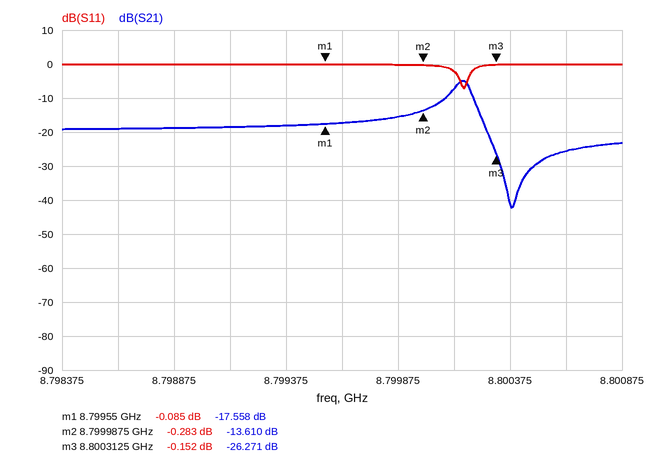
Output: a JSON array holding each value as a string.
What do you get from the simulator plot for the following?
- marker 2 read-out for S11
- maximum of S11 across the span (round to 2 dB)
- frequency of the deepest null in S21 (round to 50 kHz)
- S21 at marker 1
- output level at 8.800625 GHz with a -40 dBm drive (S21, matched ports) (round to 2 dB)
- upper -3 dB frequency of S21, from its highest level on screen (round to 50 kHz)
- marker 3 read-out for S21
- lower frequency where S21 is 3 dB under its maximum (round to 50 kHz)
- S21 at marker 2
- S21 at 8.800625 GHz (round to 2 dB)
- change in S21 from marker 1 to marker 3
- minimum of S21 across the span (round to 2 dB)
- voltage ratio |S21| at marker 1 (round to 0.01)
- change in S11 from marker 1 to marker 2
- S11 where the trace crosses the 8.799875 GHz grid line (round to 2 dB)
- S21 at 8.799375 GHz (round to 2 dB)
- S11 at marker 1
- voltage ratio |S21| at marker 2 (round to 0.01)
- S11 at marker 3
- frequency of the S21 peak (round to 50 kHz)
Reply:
["-0.283 dB", "0 dB", "8.80040 GHz", "-17.558 dB", "-66 dBm", "8.80020 GHz", "-26.271 dB", "8.80010 GHz", "-13.610 dB", "-26 dB", "-8.713 dB", "-42 dB", "0.13", "-0.198 dB", "0 dB", "-18 dB", "-0.085 dB", "0.21", "-0.152 dB", "8.80015 GHz"]
